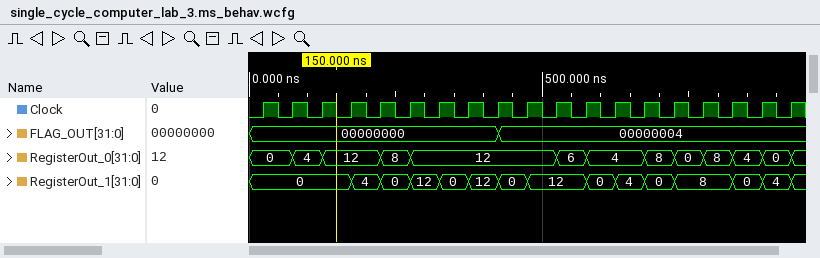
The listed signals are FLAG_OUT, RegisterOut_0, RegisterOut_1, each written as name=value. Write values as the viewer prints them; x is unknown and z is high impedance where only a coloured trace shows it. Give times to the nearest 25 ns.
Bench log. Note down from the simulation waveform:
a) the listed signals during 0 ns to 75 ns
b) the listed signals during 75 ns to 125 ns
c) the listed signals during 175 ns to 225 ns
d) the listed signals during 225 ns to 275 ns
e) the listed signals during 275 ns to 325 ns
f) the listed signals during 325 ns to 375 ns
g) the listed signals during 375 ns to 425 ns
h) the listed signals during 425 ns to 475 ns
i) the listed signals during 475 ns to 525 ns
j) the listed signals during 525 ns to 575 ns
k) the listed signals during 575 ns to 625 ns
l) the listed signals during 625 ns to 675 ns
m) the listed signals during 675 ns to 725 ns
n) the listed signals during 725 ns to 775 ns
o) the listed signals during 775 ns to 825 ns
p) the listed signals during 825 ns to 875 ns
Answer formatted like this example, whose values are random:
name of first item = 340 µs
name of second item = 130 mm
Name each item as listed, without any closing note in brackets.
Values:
the listed signals during 0 ns to 75 ns = FLAG_OUT=00000000, RegisterOut_0=0, RegisterOut_1=0
the listed signals during 75 ns to 125 ns = FLAG_OUT=00000000, RegisterOut_0=4, RegisterOut_1=0
the listed signals during 175 ns to 225 ns = FLAG_OUT=00000000, RegisterOut_0=12, RegisterOut_1=4
the listed signals during 225 ns to 275 ns = FLAG_OUT=00000000, RegisterOut_0=8, RegisterOut_1=0
the listed signals during 275 ns to 325 ns = FLAG_OUT=00000000, RegisterOut_0=12, RegisterOut_1=12
the listed signals during 325 ns to 375 ns = FLAG_OUT=00000000, RegisterOut_0=12, RegisterOut_1=0
the listed signals during 375 ns to 425 ns = FLAG_OUT=00000000, RegisterOut_0=12, RegisterOut_1=12
the listed signals during 425 ns to 475 ns = FLAG_OUT=00000004, RegisterOut_0=12, RegisterOut_1=0
the listed signals during 475 ns to 525 ns = FLAG_OUT=00000004, RegisterOut_0=12, RegisterOut_1=12
the listed signals during 525 ns to 575 ns = FLAG_OUT=00000004, RegisterOut_0=6, RegisterOut_1=12
the listed signals during 575 ns to 625 ns = FLAG_OUT=00000004, RegisterOut_0=4, RegisterOut_1=0
the listed signals during 625 ns to 675 ns = FLAG_OUT=00000004, RegisterOut_0=4, RegisterOut_1=4
the listed signals during 675 ns to 725 ns = FLAG_OUT=00000004, RegisterOut_0=8, RegisterOut_1=0
the listed signals during 725 ns to 775 ns = FLAG_OUT=00000004, RegisterOut_0=0, RegisterOut_1=8
the listed signals during 775 ns to 825 ns = FLAG_OUT=00000004, RegisterOut_0=8, RegisterOut_1=8
the listed signals during 825 ns to 875 ns = FLAG_OUT=00000004, RegisterOut_0=4, RegisterOut_1=0
